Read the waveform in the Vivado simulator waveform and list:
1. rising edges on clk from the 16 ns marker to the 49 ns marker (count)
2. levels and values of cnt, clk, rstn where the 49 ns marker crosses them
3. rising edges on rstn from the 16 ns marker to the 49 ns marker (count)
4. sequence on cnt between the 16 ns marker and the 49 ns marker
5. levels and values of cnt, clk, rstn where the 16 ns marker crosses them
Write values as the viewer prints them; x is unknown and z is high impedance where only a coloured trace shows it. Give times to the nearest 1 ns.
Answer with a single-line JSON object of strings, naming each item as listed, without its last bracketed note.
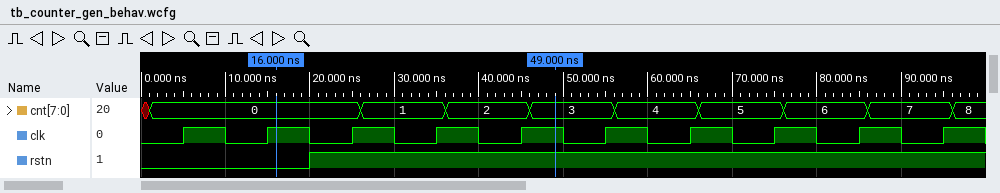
{"rising edges on clk from the 16 ns marker to the 49 ns marker": "3", "levels and values of cnt, clk, rstn where the 49 ns marker crosses them": "cnt=3, clk=1, rstn=1", "rising edges on rstn from the 16 ns marker to the 49 ns marker": "1", "sequence on cnt between the 16 ns marker and the 49 ns marker": "0, 1, 2, 3", "levels and values of cnt, clk, rstn where the 16 ns marker crosses them": "cnt=0, clk=1, rstn=0"}
